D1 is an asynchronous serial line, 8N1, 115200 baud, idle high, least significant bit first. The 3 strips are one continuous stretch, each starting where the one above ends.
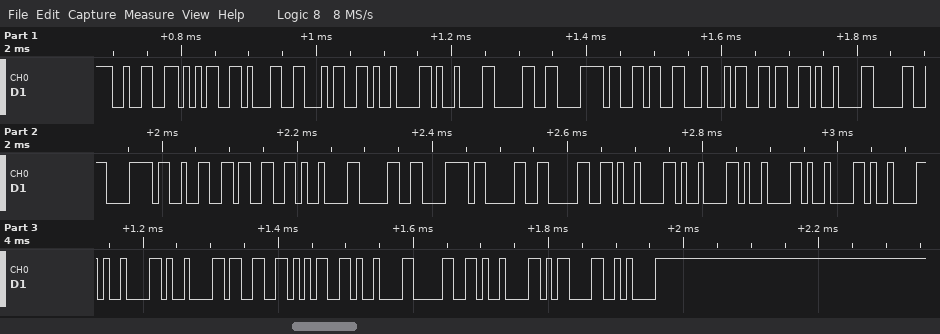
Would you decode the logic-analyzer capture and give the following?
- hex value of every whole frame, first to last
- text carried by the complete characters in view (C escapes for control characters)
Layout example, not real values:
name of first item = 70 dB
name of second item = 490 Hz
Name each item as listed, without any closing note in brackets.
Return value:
hex value of every whole frame, first to last = 0x32 0x35 0x31 0x34 0x09 0x09 0x30 0x78 0x36 0x44 0x36 0x09 0x30 0x78 0x32 0x33 0x09 0x30 0x78 0x30 0x30 0x09 0x09 0x09 0x09 0x09 0x09 0x09 0x33 0x35 0x09 0x30 0x09 0x0D 0x0A
text carried by the complete characters in view = "2514\t\t0x6D6\t0x23\t0x00\t\t\t\t\t\t\t35\t0\t\r\n"
